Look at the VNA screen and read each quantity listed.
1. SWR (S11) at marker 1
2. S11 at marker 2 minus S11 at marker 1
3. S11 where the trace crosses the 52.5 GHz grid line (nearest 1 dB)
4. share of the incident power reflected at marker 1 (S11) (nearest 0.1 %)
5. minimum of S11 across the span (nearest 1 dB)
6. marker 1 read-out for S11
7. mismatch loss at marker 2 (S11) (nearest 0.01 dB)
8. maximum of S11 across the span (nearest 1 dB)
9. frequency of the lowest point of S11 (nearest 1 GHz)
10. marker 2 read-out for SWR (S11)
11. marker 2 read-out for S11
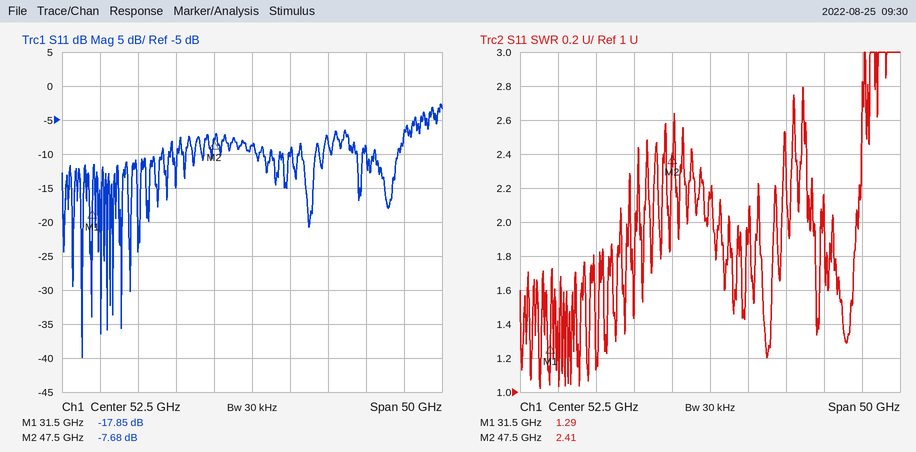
1.29
10.17 dB
-9 dB
1.6 %
-40 dB
-17.85 dB
0.81 dB
-3 dB
30 GHz
2.41
-7.68 dB
